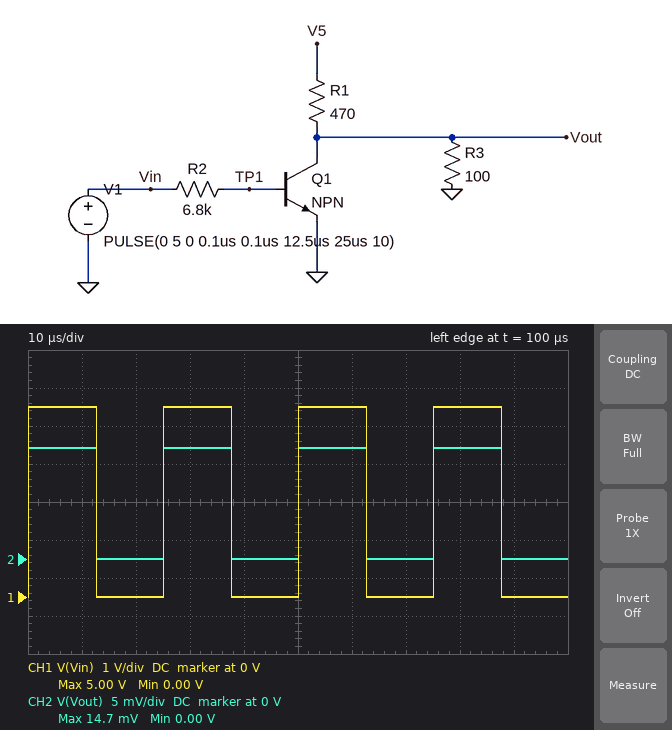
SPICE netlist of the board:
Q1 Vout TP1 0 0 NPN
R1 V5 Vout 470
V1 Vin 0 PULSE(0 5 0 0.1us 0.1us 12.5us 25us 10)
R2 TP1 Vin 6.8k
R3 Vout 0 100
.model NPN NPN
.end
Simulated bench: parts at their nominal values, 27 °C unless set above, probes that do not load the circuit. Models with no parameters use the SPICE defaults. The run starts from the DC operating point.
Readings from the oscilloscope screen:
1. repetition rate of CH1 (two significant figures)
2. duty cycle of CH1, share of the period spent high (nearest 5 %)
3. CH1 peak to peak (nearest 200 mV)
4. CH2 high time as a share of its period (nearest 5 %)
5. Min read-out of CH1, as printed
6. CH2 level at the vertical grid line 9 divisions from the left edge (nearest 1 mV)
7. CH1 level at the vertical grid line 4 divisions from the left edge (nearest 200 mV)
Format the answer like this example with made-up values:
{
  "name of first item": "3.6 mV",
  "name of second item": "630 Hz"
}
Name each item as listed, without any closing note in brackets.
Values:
{
  "repetition rate of CH1": "40 kHz",
  "duty cycle of CH1, share of the period spent high": "50 %",
  "CH1 peak to peak": "5.0 V",
  "CH2 high time as a share of its period": "50 %",
  "Min read-out of CH1, as printed": "0.00 V",
  "CH2 level at the vertical grid line 9 divisions from the left edge": "0 V",
  "CH1 level at the vertical grid line 4 divisions from the left edge": "0 V"
}
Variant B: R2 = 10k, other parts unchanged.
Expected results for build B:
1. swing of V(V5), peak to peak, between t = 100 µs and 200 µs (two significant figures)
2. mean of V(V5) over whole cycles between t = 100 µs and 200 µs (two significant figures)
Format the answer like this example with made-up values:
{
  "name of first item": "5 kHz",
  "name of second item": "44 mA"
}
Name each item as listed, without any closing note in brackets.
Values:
{
  "swing of V(V5), peak to peak, between t = 100 µs and 200 µs": "13 mV",
  "mean of V(V5) over whole cycles between t = 100 µs and 200 µs": "6.8 mV"
}
